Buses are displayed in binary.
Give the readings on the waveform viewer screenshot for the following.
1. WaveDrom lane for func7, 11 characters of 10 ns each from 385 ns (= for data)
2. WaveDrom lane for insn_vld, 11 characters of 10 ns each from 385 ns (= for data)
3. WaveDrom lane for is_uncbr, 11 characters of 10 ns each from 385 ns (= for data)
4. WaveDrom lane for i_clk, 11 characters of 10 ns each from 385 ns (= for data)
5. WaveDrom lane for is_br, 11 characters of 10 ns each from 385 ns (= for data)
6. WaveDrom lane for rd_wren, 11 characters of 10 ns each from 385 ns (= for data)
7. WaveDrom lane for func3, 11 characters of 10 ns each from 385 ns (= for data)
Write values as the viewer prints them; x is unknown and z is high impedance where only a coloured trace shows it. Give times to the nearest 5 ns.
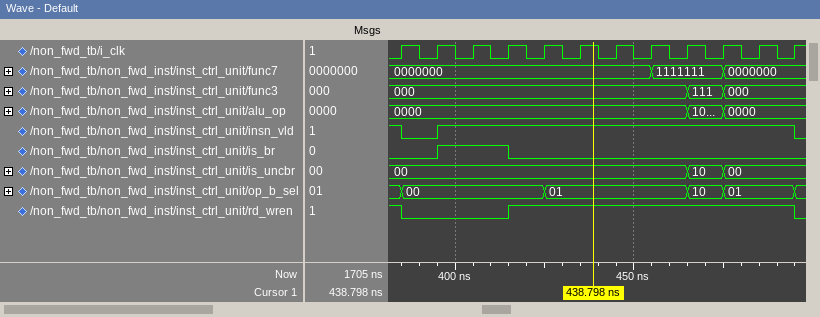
{name: 'func7', wave: '=......=.=.', data: '0000000 1111111 0000000'}
{name: 'insn_vld', wave: '01.........'}
{name: 'is_uncbr', wave: '=.......==.', data: '00 10 00'}
{name: 'i_clk', wave: 'p..........'}
{name: 'is_br', wave: '01.0.......'}
{name: 'rd_wren', wave: '0..1.......'}
{name: 'func3', wave: '=.......==.', data: '000 111 000'}
